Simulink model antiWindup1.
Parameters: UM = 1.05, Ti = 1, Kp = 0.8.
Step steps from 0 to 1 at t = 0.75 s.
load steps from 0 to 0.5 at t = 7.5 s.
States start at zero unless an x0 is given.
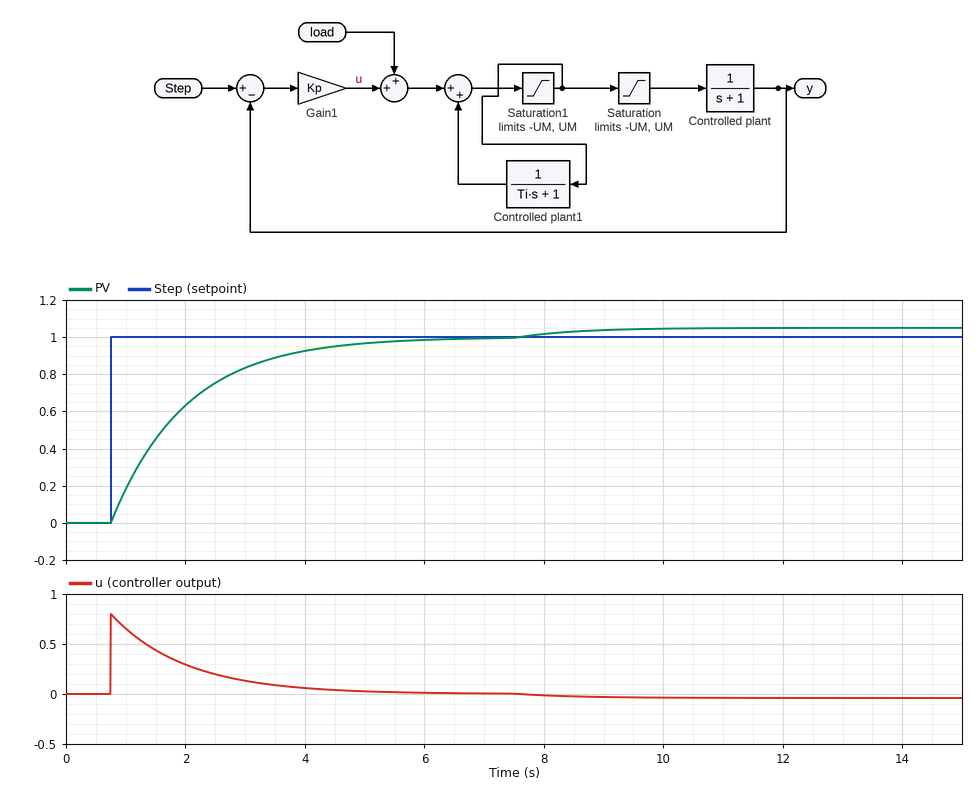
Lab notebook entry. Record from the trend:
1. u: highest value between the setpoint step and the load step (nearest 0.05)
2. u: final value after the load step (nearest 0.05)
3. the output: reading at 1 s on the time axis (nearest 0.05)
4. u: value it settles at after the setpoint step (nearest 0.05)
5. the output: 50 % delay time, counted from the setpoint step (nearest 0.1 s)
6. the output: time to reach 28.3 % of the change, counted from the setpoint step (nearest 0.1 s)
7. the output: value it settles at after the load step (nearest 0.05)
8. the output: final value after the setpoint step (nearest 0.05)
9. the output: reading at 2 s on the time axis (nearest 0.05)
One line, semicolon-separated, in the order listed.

0.80; -0.05; 0.20; 0.00; 0.9 s; 0.4 s; 1.05; 1.00; 0.65
